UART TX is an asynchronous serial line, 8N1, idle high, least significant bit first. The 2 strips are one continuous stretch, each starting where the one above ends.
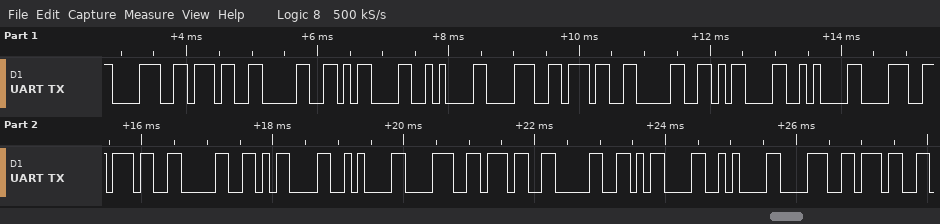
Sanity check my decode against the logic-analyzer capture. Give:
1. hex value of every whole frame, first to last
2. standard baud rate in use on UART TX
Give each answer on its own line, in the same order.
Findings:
0x38 0x37 0x30 0x0D 0x0A 0x38 0x37 0x30 0x0D 0x0A 0x38 0x37 0x30 0x0D 0x0A 0x38 0x37 0x30 0x0D 0x0A 0x38 0x37
9600 baud
